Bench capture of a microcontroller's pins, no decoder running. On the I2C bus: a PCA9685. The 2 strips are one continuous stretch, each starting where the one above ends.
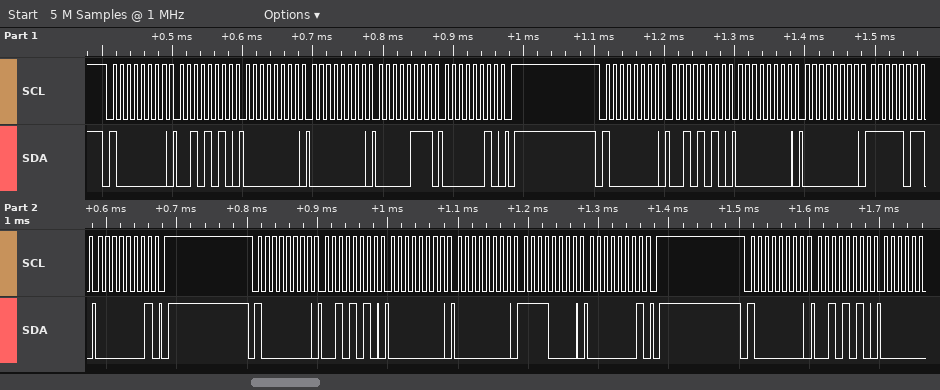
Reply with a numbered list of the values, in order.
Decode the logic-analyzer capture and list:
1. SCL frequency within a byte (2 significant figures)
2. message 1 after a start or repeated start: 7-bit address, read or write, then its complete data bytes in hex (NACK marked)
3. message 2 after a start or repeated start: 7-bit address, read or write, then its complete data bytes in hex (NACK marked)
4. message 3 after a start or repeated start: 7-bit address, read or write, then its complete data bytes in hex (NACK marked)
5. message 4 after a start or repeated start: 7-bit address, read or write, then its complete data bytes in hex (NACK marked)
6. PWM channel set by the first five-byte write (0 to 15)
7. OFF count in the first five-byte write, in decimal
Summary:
1. 100 kHz
2. 0x40 write: 2A 00 00 07 02
3. 0x40 write: 2A 00 00 FB 01
4. 0x40 write: 2A 00 00 F0 01
5. 0x40 write: 2A
6. 9
7. 519
